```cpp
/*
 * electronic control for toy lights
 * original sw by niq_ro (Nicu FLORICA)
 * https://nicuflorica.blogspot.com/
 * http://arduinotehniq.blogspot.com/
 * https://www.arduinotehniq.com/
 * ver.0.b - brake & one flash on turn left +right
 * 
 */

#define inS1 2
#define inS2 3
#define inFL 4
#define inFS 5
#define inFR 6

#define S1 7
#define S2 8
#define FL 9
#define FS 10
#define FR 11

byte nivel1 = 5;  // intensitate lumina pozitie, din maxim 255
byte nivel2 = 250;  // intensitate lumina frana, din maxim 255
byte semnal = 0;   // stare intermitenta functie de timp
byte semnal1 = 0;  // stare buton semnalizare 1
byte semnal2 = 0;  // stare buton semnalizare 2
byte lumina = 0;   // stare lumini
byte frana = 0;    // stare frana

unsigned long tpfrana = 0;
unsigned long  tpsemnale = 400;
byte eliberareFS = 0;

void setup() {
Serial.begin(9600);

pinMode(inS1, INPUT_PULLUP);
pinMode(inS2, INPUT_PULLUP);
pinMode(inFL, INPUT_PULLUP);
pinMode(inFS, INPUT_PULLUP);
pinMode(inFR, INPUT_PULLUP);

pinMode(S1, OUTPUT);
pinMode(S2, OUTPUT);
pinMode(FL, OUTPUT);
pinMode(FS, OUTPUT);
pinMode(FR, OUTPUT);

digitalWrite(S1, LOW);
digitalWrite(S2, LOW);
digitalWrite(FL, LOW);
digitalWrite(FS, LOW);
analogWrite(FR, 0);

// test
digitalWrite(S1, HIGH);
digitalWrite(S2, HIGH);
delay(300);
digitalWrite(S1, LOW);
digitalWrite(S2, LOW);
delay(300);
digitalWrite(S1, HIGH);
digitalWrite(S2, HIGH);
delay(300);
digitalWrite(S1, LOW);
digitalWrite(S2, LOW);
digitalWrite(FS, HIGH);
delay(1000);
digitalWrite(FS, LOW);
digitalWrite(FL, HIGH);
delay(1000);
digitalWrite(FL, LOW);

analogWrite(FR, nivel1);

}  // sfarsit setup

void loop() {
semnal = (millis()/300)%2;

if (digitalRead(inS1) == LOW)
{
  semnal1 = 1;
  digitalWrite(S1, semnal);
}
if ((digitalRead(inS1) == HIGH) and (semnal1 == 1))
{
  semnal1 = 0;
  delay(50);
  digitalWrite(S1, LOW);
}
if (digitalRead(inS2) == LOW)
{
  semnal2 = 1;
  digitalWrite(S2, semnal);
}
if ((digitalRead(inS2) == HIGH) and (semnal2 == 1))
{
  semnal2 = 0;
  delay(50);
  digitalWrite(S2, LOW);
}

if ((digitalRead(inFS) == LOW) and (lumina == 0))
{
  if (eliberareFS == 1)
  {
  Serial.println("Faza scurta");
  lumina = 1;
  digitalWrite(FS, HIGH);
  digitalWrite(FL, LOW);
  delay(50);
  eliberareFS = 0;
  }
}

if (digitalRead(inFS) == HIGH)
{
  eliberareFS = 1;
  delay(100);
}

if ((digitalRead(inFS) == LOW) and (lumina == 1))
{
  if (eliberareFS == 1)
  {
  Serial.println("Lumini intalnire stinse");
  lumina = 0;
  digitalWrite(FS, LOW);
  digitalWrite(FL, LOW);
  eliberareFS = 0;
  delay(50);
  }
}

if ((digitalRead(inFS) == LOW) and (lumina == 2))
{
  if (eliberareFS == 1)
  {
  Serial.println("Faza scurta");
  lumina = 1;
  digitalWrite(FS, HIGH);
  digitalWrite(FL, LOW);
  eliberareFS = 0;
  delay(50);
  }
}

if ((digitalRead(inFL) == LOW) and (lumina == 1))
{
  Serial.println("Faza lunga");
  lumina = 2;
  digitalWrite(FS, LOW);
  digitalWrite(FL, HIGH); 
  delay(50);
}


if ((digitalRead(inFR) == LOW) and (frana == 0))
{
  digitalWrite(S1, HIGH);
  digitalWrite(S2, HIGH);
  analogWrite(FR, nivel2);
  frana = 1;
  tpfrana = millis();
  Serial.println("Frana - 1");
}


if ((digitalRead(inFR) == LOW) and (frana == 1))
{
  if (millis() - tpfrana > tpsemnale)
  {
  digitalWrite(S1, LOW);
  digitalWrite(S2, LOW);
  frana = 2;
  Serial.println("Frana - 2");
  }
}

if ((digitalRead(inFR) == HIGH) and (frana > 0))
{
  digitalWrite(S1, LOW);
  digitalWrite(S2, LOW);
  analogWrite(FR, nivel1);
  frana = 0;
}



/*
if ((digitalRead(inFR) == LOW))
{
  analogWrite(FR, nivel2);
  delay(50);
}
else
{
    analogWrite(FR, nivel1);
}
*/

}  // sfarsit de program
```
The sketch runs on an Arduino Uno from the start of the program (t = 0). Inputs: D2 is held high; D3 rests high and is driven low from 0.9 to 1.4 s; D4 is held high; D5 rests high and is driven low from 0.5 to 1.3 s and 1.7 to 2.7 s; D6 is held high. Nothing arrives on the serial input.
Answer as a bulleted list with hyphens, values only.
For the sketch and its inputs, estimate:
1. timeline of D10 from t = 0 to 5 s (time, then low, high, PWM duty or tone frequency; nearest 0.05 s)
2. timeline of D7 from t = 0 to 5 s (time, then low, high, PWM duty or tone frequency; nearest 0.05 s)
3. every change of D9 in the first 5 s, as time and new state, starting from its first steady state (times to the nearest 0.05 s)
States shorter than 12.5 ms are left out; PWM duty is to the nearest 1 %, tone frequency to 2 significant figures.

- 0 s low; 0.9 s high; 1.9 s low
- 0 s high; 0.3 s low; 0.6 s high; 0.9 s low
- 0 s low; 1.9 s high; 2.9 s low
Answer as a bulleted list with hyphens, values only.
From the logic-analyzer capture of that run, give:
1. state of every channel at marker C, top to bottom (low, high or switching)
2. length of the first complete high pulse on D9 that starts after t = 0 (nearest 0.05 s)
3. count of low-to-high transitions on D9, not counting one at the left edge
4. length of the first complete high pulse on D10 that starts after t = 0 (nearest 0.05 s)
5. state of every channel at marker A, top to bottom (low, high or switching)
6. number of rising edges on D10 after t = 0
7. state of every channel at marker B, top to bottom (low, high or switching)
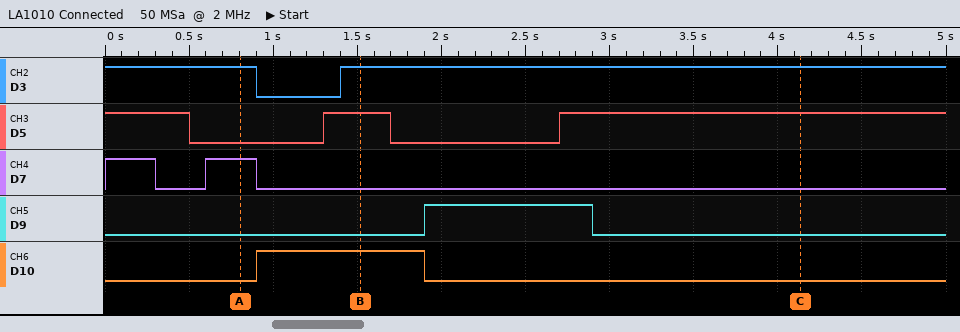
- D3 high, D5 high, D7 low, D9 low, D10 low
- 1.00 s
- 1
- 1.00 s
- D3 high, D5 low, D7 high, D9 low, D10 low
- 1
- D3 high, D5 high, D7 low, D9 low, D10 high
